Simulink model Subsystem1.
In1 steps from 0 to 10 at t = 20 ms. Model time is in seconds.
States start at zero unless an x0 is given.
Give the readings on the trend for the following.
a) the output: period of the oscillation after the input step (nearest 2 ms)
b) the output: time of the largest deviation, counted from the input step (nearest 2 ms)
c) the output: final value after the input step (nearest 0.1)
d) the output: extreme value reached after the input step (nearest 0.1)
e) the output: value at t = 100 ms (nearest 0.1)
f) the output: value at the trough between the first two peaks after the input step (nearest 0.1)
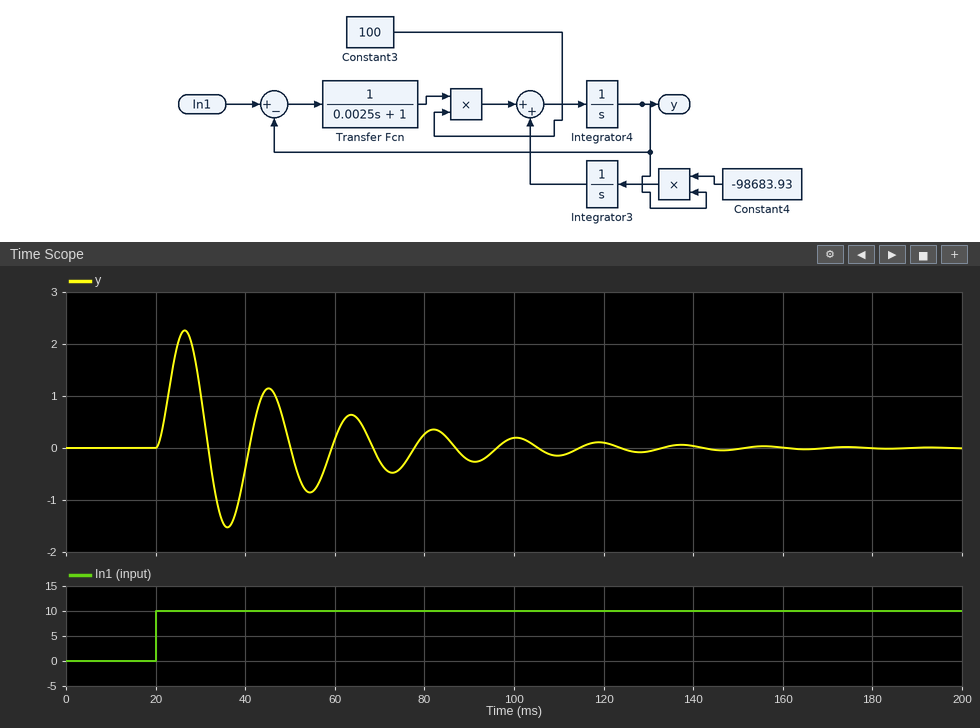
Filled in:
18 ms
6 ms
0.0
2.3
0.2
-1.5
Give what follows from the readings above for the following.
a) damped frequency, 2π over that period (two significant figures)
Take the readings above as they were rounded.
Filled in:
0.35 rad/ms
